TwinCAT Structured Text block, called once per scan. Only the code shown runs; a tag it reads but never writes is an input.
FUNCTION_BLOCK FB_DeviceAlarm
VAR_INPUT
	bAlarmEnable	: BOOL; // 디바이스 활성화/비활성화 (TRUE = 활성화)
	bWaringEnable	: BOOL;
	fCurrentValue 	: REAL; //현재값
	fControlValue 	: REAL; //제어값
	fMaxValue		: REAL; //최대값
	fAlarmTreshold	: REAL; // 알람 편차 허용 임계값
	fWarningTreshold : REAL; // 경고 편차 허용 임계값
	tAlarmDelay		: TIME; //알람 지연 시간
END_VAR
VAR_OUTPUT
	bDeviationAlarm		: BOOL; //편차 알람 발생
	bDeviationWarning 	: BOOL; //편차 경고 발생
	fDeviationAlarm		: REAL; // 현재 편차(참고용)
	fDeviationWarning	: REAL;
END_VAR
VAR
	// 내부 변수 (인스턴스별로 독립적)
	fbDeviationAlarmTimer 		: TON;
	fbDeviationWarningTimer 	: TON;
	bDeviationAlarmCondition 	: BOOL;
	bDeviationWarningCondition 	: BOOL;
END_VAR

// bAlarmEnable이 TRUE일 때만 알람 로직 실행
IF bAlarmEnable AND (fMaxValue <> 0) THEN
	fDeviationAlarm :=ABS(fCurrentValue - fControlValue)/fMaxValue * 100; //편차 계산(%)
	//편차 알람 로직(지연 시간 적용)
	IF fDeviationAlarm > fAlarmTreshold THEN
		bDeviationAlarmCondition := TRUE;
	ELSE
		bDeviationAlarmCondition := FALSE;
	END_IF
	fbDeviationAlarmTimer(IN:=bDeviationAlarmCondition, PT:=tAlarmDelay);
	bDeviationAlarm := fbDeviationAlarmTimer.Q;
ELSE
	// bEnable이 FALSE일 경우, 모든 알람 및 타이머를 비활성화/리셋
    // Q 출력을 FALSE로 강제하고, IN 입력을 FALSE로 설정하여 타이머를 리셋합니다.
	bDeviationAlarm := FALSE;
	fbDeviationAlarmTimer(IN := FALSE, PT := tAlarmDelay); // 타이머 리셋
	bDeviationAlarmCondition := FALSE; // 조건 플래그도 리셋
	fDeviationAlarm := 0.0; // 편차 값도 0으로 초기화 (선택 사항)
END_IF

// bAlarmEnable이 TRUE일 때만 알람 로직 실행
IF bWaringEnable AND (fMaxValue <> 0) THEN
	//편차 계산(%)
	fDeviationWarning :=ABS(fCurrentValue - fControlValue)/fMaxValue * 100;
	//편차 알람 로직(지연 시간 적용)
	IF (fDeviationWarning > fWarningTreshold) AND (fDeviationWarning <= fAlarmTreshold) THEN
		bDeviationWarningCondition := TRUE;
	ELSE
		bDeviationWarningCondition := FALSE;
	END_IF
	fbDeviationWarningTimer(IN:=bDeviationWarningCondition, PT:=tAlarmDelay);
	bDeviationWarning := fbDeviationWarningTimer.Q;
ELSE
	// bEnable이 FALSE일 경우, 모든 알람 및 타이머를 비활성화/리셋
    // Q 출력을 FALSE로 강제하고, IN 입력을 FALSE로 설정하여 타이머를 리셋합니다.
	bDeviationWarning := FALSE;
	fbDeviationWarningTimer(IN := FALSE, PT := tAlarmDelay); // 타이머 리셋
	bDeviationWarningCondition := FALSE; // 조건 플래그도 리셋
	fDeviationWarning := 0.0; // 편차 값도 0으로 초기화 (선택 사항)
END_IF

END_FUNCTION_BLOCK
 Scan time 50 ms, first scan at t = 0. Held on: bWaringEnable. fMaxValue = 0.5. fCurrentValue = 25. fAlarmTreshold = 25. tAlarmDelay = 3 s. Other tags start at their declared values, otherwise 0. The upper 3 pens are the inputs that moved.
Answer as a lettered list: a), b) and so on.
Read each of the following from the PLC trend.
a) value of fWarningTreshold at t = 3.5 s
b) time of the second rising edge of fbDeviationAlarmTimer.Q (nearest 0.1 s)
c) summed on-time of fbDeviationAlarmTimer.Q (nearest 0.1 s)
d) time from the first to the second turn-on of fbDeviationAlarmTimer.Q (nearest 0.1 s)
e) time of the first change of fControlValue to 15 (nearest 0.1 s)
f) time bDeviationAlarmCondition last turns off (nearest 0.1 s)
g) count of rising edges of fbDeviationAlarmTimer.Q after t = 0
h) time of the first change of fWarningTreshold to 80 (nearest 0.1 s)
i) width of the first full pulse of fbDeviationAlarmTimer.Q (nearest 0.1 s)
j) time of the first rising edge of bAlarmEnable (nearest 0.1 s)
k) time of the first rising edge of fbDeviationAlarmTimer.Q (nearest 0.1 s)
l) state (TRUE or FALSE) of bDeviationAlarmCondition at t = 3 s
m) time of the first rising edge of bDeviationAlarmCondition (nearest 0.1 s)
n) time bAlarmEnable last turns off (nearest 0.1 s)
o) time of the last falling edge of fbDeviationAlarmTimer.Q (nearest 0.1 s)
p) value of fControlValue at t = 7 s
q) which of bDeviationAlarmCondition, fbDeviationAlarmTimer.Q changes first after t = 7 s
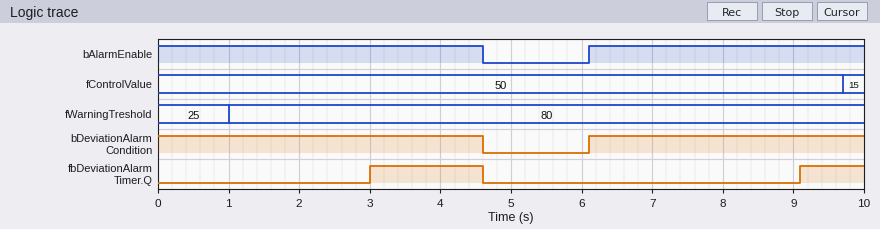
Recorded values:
a) 80
b) 9.1 s
c) 2.5 s
d) 6.1 s
e) 9.7 s
f) 4.6 s
g) 2
h) 1.0 s
i) 1.6 s
j) 6.1 s
k) 3.0 s
l) TRUE
m) 6.1 s
n) 4.6 s
o) 4.6 s
p) 50
q) fbDeviationAlarmTimer.Q
